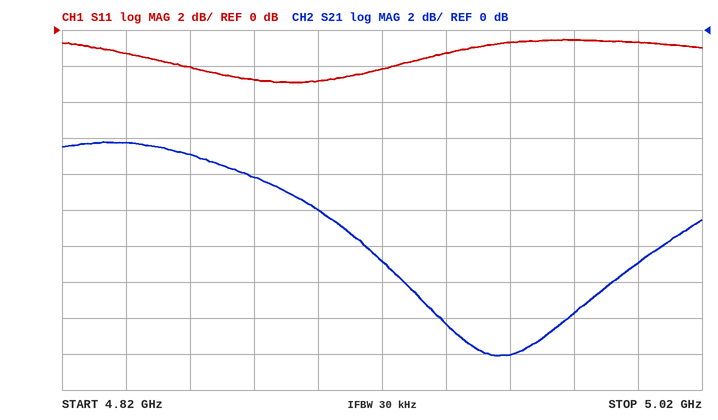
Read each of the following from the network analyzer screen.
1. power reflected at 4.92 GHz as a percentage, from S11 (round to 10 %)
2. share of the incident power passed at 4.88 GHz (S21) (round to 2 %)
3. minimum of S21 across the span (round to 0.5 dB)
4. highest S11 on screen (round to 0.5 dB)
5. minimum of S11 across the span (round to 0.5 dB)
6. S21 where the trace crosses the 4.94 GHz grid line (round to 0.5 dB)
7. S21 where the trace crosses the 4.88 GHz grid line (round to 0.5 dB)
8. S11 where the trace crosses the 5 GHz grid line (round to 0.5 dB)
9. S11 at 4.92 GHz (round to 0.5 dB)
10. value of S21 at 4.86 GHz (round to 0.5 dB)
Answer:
60 %
16 %
-18.0 dB
-0.5 dB
-3.0 dB
-16.5 dB
-8.0 dB
-0.5 dB
-2.0 dB
-7.0 dB
